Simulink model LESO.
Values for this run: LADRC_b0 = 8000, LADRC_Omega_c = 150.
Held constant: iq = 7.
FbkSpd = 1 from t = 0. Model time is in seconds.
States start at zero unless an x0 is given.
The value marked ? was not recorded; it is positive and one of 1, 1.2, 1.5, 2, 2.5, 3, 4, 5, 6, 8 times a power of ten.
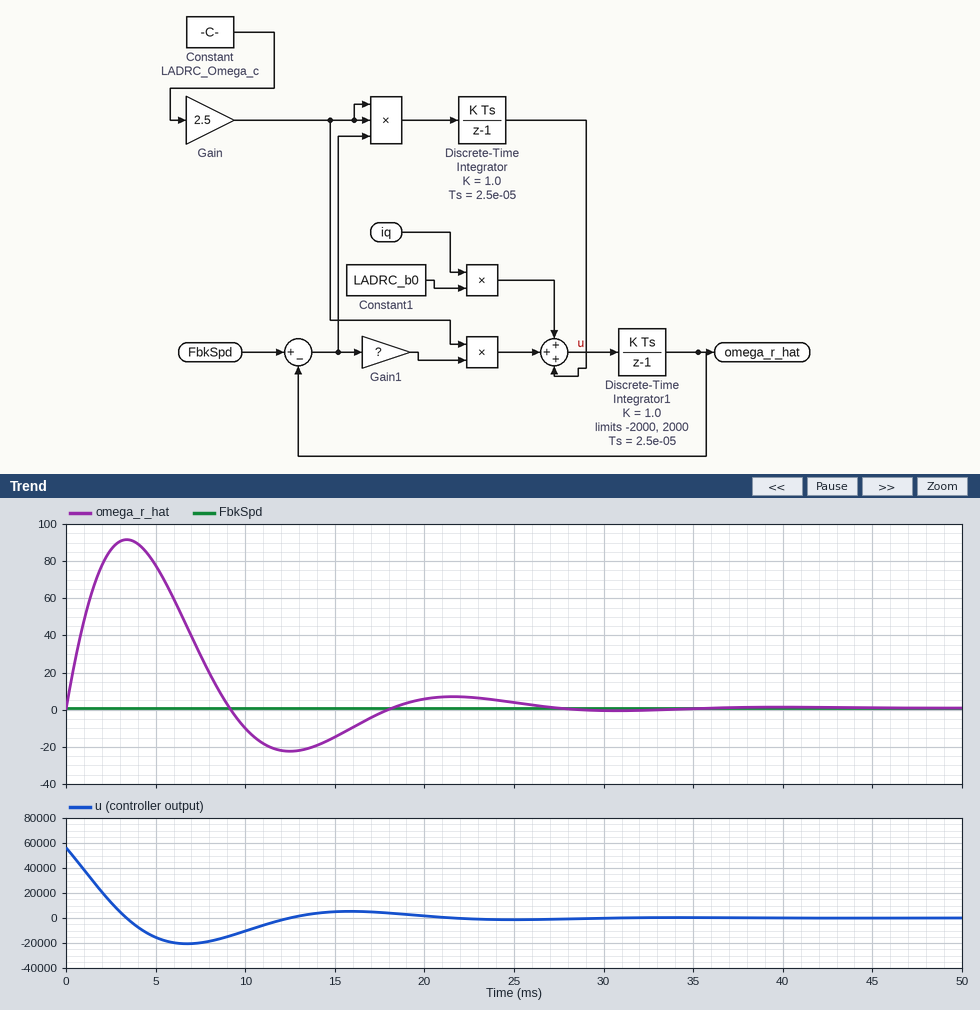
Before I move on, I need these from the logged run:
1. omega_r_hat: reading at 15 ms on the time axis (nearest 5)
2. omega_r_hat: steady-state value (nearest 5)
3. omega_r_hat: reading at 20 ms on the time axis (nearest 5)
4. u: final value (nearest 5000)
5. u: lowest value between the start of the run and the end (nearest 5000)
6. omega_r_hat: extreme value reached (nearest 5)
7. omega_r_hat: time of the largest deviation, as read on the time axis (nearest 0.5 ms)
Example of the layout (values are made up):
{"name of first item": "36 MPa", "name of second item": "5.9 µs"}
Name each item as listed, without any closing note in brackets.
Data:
{"omega_r_hat: reading at 15 ms on the time axis": "-15", "omega_r_hat: steady-state value": "0", "omega_r_hat: reading at 20 ms on the time axis": "5", "u: final value": "0", "u: lowest value between the start of the run and the end": "-20000", "omega_r_hat: extreme value reached": "90", "omega_r_hat: time of the largest deviation, as read on the time axis": "3.5 ms"}
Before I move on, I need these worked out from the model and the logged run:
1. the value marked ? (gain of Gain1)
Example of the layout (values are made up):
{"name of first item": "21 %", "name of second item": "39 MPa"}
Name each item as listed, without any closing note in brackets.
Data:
{"the value marked ?": "0.8"}
